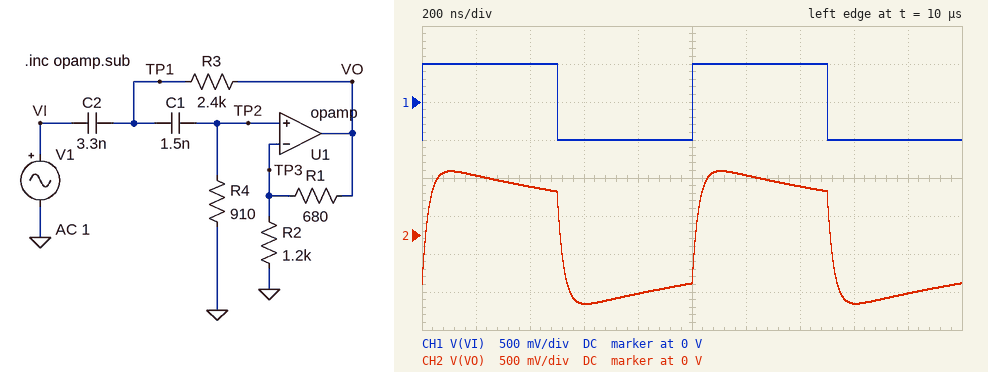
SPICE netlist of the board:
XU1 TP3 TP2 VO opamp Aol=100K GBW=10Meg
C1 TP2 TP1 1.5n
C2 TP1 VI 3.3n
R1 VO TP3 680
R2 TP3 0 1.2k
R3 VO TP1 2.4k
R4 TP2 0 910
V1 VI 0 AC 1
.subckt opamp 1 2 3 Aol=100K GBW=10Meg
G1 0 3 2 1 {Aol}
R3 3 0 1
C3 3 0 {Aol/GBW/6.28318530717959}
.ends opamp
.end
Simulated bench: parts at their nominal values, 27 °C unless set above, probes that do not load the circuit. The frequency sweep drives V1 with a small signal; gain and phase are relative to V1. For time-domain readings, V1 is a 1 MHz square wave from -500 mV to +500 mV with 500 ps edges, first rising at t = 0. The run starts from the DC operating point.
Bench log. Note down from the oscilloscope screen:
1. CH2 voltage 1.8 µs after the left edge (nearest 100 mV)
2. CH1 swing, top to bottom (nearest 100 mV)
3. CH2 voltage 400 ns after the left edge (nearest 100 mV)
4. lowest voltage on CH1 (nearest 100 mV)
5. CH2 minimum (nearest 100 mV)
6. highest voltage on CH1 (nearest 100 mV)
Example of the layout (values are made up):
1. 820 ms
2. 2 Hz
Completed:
1. -800 mV
2. 1.0 V
3. 600 mV
4. -500 mV
5. -900 mV
6. 500 mV
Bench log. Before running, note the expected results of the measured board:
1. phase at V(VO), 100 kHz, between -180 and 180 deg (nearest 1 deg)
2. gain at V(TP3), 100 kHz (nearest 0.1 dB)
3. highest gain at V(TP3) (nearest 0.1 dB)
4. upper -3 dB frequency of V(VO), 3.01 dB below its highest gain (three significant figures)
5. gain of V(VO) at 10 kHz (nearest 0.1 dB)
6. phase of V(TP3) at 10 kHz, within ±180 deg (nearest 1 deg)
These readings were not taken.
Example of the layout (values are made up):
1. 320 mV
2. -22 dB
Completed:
1. 63 deg
2. -4.9 dB
3. -0.2 dB
4. 6.69 MHz
5. -24.9 dB
6. 145 deg
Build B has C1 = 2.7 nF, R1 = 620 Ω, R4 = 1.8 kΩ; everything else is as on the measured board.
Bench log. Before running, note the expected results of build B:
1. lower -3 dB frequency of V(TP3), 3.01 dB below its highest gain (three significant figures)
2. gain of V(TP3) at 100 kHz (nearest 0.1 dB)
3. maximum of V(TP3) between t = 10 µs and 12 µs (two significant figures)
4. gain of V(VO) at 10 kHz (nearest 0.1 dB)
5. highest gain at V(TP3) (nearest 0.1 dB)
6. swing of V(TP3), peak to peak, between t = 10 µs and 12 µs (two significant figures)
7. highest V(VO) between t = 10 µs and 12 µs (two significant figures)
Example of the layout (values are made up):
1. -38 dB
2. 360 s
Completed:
1. 37.0 kHz
2. -0.5 dB
3. 450 mV
4. -13.8 dB
5. -0.1 dB
6. 1.0 V
7. 680 mV
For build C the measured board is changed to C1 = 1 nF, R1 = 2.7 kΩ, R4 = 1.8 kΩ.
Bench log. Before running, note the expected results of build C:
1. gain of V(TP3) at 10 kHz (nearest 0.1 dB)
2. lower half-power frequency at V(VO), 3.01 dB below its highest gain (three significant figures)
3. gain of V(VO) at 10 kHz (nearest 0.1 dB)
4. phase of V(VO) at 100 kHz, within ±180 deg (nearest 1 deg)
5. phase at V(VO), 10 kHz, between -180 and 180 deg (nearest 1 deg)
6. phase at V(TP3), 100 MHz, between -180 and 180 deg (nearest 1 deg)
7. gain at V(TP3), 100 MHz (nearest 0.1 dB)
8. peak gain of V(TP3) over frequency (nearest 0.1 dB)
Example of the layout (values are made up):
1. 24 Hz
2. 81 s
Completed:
1. -25.2 dB
2. 48.8 kHz
3. -14.9 dB
4. 38 deg
5. 157 deg
6. -88 deg
7. -30.2 dB
8. -0.3 dB
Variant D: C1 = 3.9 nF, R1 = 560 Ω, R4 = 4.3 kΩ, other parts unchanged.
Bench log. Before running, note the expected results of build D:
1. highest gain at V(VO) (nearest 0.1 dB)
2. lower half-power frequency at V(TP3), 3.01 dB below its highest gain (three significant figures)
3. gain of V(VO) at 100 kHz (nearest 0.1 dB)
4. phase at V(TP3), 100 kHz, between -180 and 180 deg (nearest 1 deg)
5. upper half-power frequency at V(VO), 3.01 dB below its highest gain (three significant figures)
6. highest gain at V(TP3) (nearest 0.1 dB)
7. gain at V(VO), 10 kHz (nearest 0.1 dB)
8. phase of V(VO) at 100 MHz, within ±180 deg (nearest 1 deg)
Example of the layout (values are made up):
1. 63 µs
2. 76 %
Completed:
1. 5.8 dB
2. 11.6 kHz
3. 3.4 dB
4. 6 deg
5. 2.33 MHz
6. 2.5 dB
7. 0.1 dB
8. -86 deg
